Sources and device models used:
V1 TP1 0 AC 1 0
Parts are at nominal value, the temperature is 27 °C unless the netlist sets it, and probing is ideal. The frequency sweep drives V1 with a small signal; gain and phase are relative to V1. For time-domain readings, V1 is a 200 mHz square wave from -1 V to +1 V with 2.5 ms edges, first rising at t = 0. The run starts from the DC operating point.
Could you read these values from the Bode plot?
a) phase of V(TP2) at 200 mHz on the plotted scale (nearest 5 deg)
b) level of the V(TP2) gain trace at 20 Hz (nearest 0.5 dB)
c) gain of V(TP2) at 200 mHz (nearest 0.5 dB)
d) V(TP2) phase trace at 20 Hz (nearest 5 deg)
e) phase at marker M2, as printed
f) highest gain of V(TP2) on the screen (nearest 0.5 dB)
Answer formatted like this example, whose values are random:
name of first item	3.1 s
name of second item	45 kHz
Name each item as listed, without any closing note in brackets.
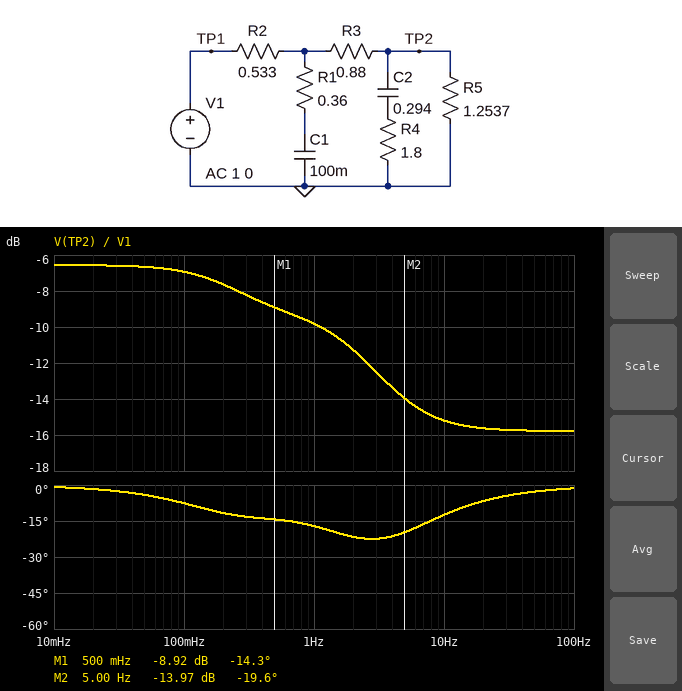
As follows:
phase of V(TP2) at 200 mHz on the plotted scale	-10 deg
level of the V(TP2) gain trace at 20 Hz	-15.5 dB
gain of V(TP2) at 200 mHz	-7.5 dB
V(TP2) phase trace at 20 Hz	-5 deg
phase at marker M2, as printed	-19.6 deg
highest gain of V(TP2) on the screen	-6.5 dB
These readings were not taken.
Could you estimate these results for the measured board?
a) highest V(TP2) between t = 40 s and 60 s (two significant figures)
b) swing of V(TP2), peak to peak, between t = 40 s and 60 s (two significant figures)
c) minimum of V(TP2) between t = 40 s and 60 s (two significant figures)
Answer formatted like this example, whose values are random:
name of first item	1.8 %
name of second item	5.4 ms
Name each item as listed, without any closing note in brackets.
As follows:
highest V(TP2) between t = 40 s and 60 s	460 mV
swing of V(TP2), peak to peak, between t = 40 s and 60 s	920 mV
minimum of V(TP2) between t = 40 s and 60 s	-460 mV
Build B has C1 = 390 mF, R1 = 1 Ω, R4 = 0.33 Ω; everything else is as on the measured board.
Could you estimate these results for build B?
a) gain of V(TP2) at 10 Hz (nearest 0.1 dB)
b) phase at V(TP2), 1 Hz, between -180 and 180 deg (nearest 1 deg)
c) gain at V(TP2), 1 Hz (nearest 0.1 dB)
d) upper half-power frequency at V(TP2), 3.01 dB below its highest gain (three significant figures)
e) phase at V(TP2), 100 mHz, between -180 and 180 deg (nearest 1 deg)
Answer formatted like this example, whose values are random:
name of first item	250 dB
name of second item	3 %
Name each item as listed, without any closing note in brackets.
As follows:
gain of V(TP2) at 10 Hz	-18.7 dB
phase at V(TP2), 1 Hz, between -180 and 180 deg	-35 deg
gain at V(TP2), 1 Hz	-14.1 dB
upper half-power frequency at V(TP2), 3.01 dB below its highest gain	360 mHz
phase at V(TP2), 100 mHz, between -180 and 180 deg	-12 deg
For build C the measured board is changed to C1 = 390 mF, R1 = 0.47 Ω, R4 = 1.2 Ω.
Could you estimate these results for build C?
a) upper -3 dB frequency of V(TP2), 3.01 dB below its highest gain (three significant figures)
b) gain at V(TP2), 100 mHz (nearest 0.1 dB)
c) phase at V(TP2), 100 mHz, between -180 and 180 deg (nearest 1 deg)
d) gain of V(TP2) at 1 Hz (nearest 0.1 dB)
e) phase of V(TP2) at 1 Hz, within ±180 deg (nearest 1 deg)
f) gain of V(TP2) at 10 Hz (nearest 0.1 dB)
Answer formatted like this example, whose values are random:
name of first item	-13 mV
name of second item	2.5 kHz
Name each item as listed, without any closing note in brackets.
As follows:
upper -3 dB frequency of V(TP2), 3.01 dB below its highest gain	331 mHz
gain at V(TP2), 100 mHz	-7.0 dB
phase at V(TP2), 100 mHz, between -180 and 180 deg	-12 deg
gain of V(TP2) at 1 Hz	-13.7 dB
phase of V(TP2) at 1 Hz, within ±180 deg	-23 deg
gain of V(TP2) at 10 Hz	-15.6 dB
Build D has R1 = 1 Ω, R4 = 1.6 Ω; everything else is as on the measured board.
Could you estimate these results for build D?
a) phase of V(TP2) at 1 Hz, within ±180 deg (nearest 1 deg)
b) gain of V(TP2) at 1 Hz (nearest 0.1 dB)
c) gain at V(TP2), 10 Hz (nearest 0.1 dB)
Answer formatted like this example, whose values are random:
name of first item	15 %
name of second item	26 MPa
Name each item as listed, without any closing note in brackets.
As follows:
phase of V(TP2) at 1 Hz, within ±180 deg	-14 deg
gain of V(TP2) at 1 Hz	-10.4 dB
gain at V(TP2), 10 Hz	-12.4 dB
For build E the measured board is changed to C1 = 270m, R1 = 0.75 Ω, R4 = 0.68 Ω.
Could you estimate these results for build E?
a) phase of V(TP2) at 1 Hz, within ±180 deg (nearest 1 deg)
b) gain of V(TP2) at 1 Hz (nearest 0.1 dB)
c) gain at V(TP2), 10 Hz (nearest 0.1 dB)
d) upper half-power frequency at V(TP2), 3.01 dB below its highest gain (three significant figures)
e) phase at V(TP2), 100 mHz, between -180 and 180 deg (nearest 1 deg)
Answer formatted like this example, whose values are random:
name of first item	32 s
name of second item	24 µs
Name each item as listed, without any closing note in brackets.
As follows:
phase of V(TP2) at 1 Hz, within ±180 deg	-27 deg
gain of V(TP2) at 1 Hz	-13.6 dB
gain at V(TP2), 10 Hz	-16.0 dB
upper half-power frequency at V(TP2), 3.01 dB below its highest gain	385 mHz
phase at V(TP2), 100 mHz, between -180 and 180 deg	-11 deg
